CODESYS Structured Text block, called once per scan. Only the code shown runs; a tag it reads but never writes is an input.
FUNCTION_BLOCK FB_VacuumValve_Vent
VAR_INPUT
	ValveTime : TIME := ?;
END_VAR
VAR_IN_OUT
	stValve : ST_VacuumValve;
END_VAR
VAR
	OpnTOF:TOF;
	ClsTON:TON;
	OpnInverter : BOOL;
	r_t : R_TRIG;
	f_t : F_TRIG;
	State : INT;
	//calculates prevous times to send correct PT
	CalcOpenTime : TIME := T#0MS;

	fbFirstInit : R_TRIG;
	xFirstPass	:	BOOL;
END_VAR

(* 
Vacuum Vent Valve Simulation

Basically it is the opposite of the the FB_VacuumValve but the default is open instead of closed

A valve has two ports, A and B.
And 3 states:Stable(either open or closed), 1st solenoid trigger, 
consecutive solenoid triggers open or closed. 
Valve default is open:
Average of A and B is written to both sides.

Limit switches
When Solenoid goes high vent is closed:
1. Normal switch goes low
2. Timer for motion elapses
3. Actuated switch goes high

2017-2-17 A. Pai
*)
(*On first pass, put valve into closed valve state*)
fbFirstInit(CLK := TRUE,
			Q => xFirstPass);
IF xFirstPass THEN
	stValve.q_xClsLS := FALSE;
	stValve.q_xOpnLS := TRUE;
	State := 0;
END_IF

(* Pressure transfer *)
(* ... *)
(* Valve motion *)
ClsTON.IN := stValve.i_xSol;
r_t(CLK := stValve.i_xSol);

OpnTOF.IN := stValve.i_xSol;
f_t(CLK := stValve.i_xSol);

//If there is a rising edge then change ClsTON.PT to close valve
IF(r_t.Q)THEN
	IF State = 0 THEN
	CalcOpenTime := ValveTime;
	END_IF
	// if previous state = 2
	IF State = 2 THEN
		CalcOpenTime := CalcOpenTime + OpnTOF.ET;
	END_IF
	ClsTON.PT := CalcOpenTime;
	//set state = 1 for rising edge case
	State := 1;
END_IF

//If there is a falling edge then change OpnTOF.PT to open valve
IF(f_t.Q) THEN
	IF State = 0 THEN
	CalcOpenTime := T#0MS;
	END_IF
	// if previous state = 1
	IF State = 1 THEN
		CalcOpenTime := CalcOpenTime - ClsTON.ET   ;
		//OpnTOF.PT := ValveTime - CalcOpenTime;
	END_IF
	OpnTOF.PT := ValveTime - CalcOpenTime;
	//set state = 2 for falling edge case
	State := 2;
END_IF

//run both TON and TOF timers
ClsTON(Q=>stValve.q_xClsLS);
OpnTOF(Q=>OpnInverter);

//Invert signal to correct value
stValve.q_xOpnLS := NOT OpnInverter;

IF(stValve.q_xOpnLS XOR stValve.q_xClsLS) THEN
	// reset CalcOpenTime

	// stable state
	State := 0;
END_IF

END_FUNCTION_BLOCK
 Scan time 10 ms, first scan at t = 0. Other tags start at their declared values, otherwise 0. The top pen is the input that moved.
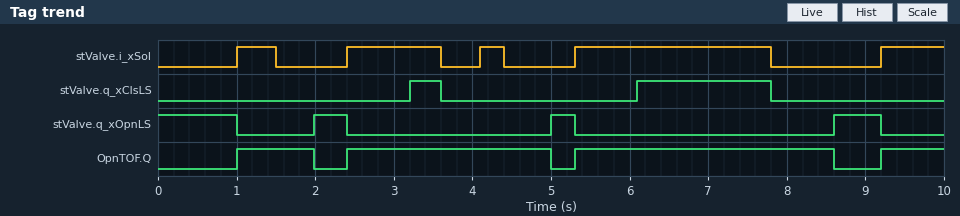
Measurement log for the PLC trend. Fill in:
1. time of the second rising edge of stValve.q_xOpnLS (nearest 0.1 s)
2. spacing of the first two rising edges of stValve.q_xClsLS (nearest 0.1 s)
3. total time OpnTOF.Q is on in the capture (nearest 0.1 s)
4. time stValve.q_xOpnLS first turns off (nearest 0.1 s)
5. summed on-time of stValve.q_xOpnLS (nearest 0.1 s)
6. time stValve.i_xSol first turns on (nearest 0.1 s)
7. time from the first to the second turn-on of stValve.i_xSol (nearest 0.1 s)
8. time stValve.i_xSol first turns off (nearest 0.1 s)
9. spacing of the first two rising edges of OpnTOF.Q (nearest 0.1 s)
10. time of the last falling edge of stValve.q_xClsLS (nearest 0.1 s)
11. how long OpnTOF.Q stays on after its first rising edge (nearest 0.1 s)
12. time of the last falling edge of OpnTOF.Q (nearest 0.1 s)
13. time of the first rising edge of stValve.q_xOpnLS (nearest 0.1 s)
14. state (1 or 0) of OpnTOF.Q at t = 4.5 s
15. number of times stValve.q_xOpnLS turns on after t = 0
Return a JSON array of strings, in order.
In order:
["5.0 s", "2.9 s", "7.7 s", "1.0 s", "2.3 s", "1.0 s", "1.4 s", "1.5 s", "1.4 s", "7.8 s", "1.0 s", "8.6 s", "2.0 s", "1", "3"]
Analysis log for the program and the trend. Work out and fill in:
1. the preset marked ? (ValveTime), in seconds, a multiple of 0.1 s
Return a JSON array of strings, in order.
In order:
["0.8 s"]
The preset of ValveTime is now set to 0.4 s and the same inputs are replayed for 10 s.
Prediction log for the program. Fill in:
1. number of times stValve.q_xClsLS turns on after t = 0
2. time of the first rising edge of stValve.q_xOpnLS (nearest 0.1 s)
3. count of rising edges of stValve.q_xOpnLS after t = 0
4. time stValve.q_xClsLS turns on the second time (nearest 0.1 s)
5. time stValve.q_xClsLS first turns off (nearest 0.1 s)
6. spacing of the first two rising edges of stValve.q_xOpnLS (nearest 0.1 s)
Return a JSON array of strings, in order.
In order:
["4", "1.9 s", "4", "2.8 s", "1.5 s", "2.1 s"]
